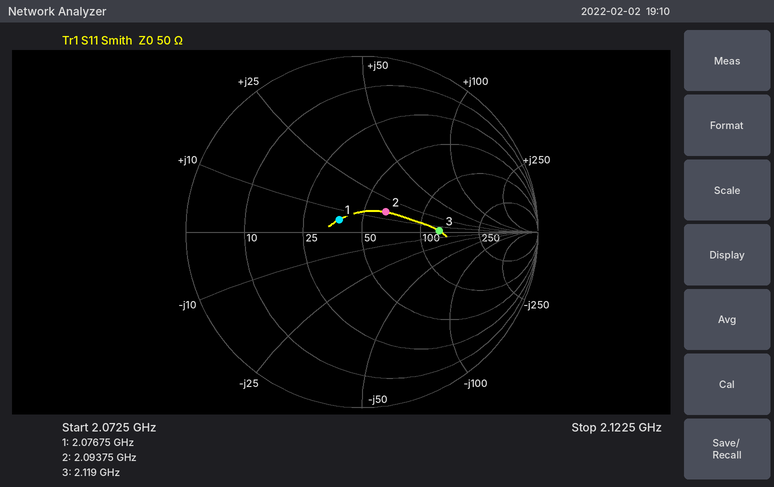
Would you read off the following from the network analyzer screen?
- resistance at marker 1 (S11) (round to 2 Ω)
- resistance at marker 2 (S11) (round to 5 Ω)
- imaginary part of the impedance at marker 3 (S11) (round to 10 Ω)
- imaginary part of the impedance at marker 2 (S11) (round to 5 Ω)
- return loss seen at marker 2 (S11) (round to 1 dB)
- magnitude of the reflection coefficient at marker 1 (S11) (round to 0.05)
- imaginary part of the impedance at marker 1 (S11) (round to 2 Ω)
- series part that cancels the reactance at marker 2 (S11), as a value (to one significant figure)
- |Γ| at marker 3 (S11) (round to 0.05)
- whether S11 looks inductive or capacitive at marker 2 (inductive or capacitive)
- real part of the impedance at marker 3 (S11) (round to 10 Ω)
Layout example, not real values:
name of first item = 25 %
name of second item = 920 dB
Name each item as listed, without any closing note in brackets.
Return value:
resistance at marker 1 (S11) = 38 Ω
resistance at marker 2 (S11) = 65 Ω
imaginary part of the impedance at marker 3 (S11) = 0 Ω
imaginary part of the impedance at marker 2 (S11) = +15 Ω
return loss seen at marker 2 (S11) = 15 dB
magnitude of the reflection coefficient at marker 1 (S11) = 0.15
imaginary part of the impedance at marker 1 (S11) = +6 Ω
series part that cancels the reactance at marker 2 (S11), as a value = 5 pF
|Γ| at marker 3 (S11) = 0.45
whether S11 looks inductive or capacitive at marker 2 = inductive
real part of the impedance at marker 3 (S11) = 130 Ω
